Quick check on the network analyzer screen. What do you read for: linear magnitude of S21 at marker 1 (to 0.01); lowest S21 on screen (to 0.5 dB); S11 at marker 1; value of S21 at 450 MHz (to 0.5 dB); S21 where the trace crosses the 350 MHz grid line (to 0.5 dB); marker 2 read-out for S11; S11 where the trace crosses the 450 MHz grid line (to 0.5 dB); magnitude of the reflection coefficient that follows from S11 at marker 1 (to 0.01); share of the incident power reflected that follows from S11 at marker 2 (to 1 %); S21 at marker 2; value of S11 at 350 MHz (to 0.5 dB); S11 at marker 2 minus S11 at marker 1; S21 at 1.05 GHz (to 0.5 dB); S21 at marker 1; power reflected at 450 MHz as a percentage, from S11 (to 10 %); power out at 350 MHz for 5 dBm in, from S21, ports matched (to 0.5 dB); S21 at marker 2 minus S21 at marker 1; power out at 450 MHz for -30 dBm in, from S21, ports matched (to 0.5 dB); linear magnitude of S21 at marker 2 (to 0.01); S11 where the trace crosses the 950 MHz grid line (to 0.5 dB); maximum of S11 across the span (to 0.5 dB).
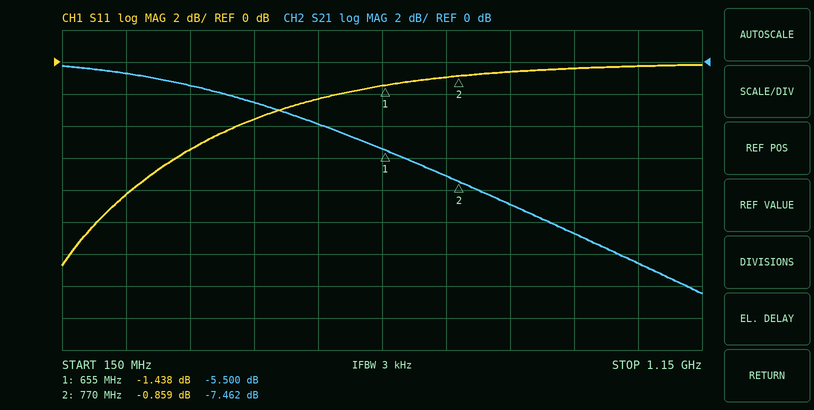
0.53
-14.5 dB
-1.438 dB
-2.5 dB
-1.5 dB
-0.859 dB
-3.5 dB
0.85
82 %
-7.462 dB
-5.5 dB
0.579 dB
-12.5 dB
-5.500 dB
40 %
3.5 dBm
-1.962 dB
-32.5 dBm
0.42
-0.5 dB
0.0 dB
